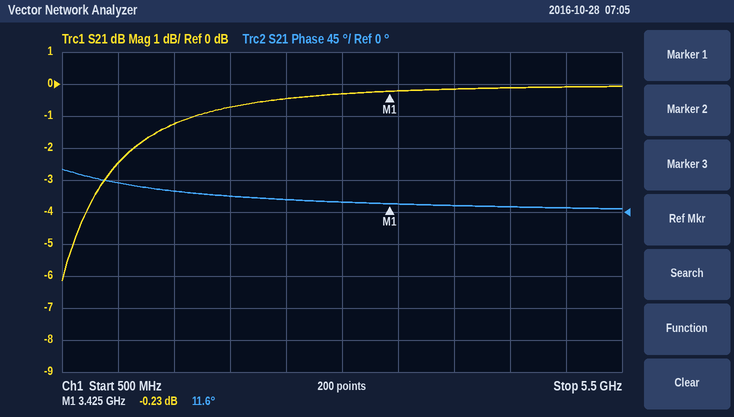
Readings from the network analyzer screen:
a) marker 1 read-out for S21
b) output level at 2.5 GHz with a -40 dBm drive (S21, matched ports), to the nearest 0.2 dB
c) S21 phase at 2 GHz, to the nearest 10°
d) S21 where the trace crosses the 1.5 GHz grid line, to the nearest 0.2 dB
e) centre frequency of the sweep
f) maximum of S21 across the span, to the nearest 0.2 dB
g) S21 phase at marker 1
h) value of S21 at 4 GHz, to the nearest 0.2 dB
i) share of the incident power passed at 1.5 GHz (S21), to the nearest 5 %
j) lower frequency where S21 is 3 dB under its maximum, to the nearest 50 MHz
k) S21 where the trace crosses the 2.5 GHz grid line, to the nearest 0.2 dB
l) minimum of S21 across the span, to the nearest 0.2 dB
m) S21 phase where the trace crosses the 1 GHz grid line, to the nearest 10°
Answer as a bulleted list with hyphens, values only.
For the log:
- -0.23 dB
- -40.4 dBm
- 20°
- -1.2 dB
- 3 GHz
- 0.0 dB
- 11.6°
- -0.2 dB
- 75 %
- 850 MHz
- -0.4 dB
- -6.2 dB
- 40°
